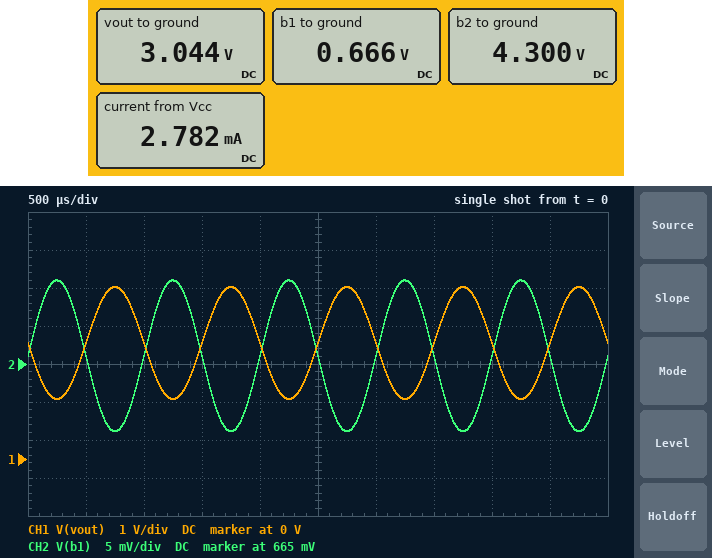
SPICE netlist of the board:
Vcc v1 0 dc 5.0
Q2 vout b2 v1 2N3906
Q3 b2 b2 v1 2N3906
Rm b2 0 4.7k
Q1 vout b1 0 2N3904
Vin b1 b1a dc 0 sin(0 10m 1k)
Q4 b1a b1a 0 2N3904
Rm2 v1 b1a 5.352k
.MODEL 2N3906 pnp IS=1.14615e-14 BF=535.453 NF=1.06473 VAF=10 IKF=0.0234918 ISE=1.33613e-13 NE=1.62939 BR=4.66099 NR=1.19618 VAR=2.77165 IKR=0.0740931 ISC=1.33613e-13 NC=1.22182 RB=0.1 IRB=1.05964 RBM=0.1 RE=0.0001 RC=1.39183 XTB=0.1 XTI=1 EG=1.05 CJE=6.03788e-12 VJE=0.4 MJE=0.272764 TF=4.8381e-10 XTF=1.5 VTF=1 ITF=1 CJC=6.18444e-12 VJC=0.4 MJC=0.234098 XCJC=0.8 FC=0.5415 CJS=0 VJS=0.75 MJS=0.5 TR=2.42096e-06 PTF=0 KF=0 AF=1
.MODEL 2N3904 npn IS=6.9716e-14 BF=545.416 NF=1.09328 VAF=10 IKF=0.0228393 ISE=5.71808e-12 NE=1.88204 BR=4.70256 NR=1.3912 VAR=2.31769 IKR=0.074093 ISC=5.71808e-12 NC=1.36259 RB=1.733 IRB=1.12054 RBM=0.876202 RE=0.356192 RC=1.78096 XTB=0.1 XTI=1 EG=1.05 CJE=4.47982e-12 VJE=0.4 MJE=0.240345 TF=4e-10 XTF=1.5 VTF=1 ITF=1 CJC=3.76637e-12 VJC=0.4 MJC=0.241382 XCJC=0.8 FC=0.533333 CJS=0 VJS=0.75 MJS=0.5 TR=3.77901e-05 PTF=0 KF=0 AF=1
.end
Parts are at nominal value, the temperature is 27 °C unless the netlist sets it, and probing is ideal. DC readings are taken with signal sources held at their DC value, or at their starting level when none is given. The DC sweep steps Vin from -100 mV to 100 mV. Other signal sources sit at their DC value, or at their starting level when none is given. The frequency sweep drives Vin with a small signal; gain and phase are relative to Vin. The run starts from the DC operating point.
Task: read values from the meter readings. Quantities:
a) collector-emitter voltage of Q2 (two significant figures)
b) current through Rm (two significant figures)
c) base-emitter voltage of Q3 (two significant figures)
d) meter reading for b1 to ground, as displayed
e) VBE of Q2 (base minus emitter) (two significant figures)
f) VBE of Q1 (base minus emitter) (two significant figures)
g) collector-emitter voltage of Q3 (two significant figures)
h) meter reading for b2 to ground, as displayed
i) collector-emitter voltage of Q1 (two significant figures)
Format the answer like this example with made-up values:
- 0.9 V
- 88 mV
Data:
- -2.0 V
- 910 µA
- -700 mV
- 0.666 V
- -700 mV
- 670 mV
- -700 mV
- 4.300 V
- 3.0 V
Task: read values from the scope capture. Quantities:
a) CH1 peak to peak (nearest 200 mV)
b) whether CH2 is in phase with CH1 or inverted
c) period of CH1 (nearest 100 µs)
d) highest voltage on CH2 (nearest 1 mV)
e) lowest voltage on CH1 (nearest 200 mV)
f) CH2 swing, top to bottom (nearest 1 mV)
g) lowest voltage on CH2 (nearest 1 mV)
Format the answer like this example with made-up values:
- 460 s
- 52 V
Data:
- 3.0 V
- inverted
- 1.0 ms
- 676 mV
- 1.6 V
- 20 mV
- 656 mV
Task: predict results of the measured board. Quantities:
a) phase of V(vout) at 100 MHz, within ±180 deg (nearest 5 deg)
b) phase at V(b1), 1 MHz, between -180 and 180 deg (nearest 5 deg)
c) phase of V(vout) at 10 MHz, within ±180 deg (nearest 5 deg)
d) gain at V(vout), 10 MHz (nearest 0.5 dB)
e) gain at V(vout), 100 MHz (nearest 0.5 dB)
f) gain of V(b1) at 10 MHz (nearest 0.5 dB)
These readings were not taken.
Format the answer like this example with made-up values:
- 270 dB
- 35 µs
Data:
- 90 deg
- -5 deg
- 105 deg
- 31.0 dB
- 11.5 dB
- -2.0 dB
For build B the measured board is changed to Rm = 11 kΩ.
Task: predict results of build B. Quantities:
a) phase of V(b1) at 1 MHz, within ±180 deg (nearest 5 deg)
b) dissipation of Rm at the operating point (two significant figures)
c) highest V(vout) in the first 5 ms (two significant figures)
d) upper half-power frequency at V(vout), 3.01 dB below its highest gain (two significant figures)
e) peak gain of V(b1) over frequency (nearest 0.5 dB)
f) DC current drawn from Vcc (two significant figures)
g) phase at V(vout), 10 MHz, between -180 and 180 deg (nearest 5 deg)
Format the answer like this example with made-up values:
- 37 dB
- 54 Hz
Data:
- 0 deg
- 1.7 mW
- 690 mV
- 510 kHz
- -5.0 dB
- 1.8 mA
- 30 deg
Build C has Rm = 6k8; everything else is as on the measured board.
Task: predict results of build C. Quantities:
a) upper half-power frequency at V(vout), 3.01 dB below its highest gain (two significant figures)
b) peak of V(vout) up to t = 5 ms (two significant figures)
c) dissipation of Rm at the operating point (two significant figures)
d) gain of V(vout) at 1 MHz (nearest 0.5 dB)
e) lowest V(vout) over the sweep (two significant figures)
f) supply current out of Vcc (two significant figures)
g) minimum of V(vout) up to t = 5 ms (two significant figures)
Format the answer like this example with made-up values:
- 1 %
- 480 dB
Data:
- 2.0 MHz
- 2.9 V
- 2.7 mW
- 42.5 dB
- 37 mV
- 2.3 mA
- 150 mV
